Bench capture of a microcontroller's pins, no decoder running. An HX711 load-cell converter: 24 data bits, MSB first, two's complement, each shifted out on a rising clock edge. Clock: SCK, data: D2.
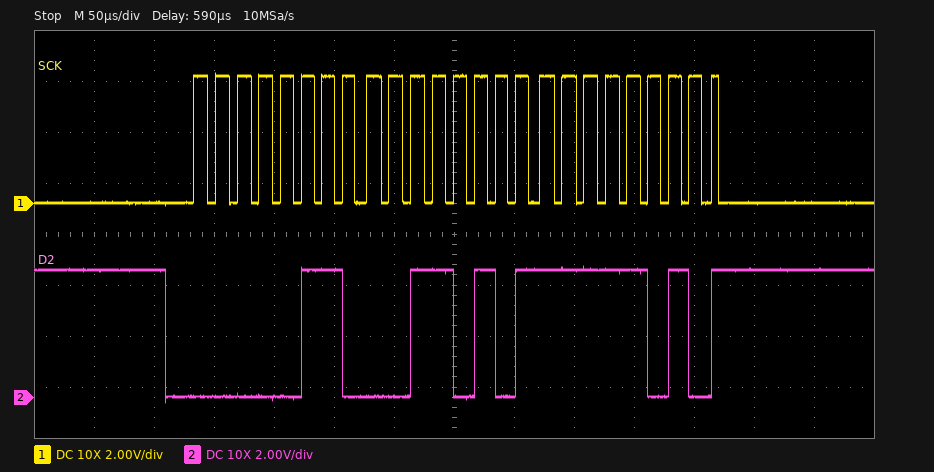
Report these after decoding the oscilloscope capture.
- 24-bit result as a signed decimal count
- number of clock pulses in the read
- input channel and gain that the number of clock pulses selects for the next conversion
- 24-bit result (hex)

407034
25
channel A, gain 128
0x0635FA
